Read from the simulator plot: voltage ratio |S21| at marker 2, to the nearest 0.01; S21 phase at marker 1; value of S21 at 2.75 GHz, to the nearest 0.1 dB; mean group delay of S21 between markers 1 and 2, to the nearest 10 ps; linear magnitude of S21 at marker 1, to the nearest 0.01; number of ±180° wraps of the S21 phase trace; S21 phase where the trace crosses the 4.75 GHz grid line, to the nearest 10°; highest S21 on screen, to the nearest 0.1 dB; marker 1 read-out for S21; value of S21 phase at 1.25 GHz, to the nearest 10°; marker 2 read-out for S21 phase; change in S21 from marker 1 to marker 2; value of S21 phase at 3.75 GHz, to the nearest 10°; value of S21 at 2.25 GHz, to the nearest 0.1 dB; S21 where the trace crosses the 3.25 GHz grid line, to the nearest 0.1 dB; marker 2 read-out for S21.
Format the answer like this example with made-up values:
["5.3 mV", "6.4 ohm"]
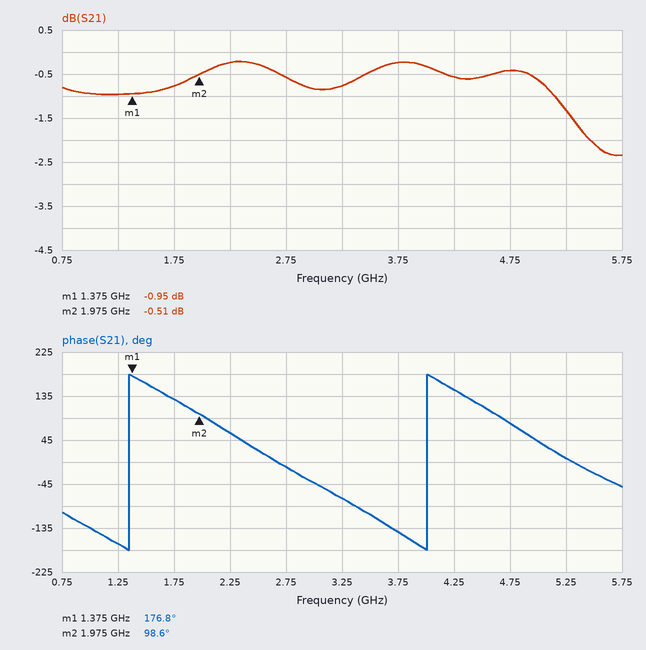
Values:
["0.94", "176.8°", "-0.6 dB", "360 ps", "0.90", "2", "80°", "-0.2 dB", "-0.95 dB", "-170°", "98.6°", "0.44 dB", "-140°", "-0.2 dB", "-0.8 dB", "-0.51 dB"]
